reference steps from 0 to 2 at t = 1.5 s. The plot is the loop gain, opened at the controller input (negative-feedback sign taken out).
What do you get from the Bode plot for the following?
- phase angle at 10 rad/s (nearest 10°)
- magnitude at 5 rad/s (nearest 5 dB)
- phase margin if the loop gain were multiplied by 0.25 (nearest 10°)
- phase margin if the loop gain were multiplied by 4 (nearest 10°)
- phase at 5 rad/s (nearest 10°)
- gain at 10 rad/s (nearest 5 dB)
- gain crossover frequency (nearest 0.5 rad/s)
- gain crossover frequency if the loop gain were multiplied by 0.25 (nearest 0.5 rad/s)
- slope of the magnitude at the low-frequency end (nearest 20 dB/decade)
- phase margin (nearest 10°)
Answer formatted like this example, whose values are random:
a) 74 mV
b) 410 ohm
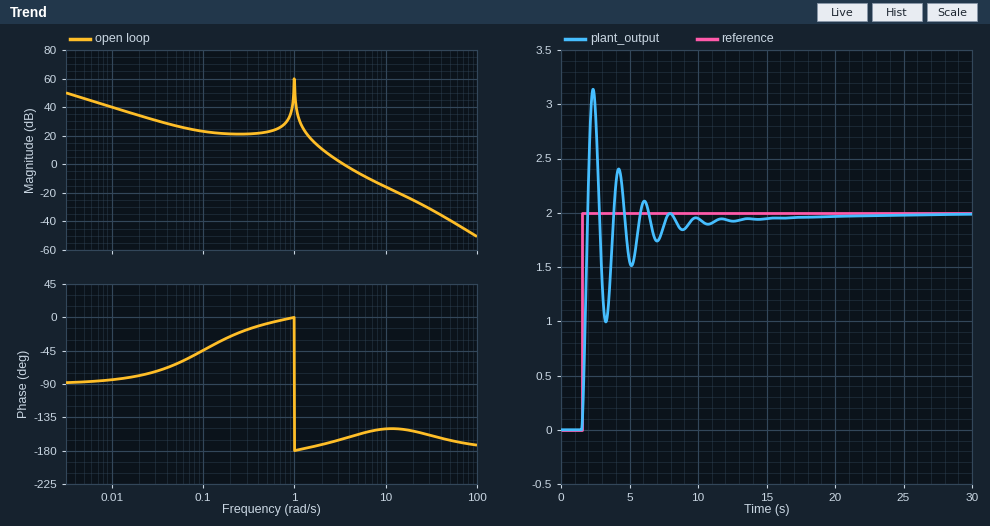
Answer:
a) -150°
b) -5 dB
c) 10°
d) 30°
e) -160°
f) -15 dB
g) 3.5 rad/s
h) 2.0 rad/s
i) -20 dB/decade
j) 20°
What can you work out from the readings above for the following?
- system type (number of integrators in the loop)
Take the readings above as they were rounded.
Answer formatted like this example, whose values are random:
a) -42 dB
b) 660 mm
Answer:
a) 1
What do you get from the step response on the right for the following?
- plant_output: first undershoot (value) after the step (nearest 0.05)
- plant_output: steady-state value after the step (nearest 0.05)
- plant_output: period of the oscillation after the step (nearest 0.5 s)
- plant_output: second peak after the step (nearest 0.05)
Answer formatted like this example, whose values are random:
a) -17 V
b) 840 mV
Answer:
a) 1.00
b) 2.00
c) 2.0 s
d) 2.40
